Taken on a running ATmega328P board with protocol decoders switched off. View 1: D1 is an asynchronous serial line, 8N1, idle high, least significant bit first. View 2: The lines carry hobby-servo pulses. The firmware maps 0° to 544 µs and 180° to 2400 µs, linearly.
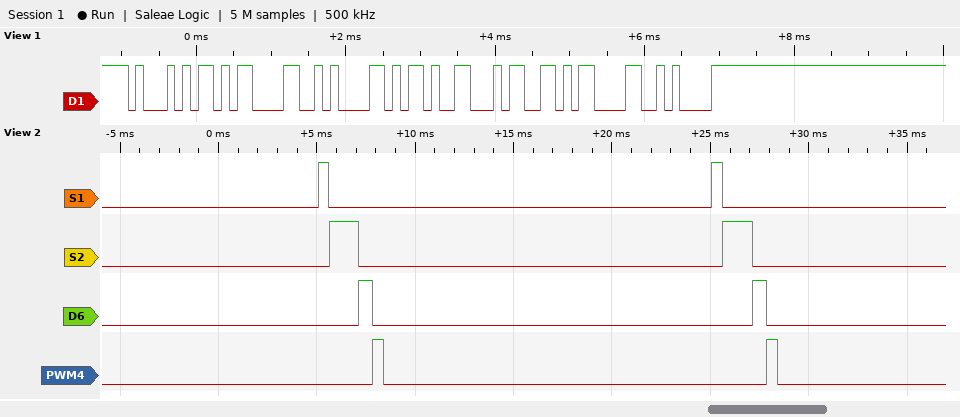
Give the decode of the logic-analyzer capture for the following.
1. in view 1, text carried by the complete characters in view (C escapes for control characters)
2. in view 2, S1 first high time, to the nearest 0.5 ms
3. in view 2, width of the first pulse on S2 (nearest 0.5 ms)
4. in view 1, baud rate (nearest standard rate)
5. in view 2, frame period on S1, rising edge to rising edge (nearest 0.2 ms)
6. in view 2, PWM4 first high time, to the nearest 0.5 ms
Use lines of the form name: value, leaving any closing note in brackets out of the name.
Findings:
in view 1, text carried by the complete characters in view: "Q\r\n-4\r\n"
in view 2, S1 first high time, to the nearest 0.5 ms: 0.5 ms
in view 2, width of the first pulse on S2: 1.5 ms
in view 1, baud rate: 9600 baud
in view 2, frame period on S1, rising edge to rising edge: 20.0 ms
in view 2, PWM4 first high time, to the nearest 0.5 ms: 0.5 ms
